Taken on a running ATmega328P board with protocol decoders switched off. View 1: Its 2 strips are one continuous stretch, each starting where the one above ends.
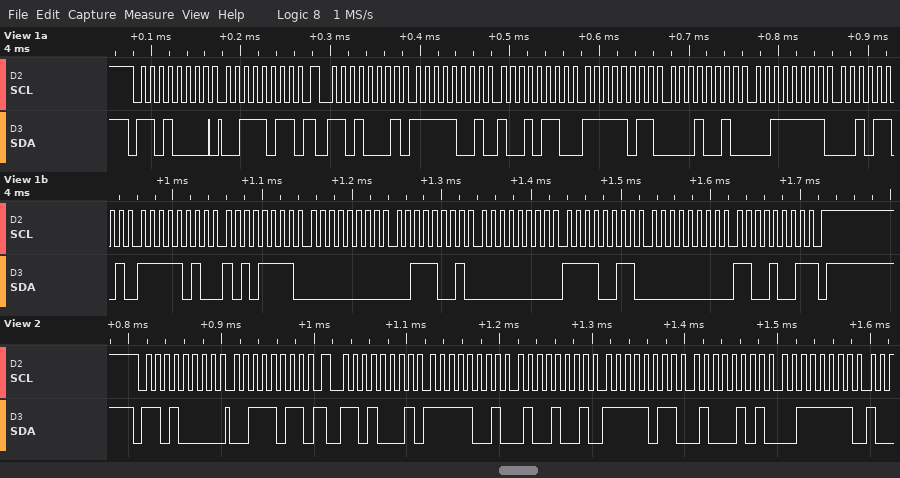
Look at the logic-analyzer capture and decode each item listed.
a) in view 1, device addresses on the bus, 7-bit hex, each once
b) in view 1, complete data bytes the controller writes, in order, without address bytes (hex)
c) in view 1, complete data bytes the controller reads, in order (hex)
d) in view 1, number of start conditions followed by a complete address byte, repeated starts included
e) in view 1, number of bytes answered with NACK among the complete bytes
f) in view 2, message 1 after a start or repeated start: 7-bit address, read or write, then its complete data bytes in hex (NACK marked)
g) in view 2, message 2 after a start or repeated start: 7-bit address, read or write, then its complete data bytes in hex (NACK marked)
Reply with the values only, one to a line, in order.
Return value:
0x68
3B
F9 96 FB 12 3F 2D FA AF 00 39 00 F3 00 C9
2
1
0x68 write: 3B
0x68 read: F9 49 FB 45 3F
